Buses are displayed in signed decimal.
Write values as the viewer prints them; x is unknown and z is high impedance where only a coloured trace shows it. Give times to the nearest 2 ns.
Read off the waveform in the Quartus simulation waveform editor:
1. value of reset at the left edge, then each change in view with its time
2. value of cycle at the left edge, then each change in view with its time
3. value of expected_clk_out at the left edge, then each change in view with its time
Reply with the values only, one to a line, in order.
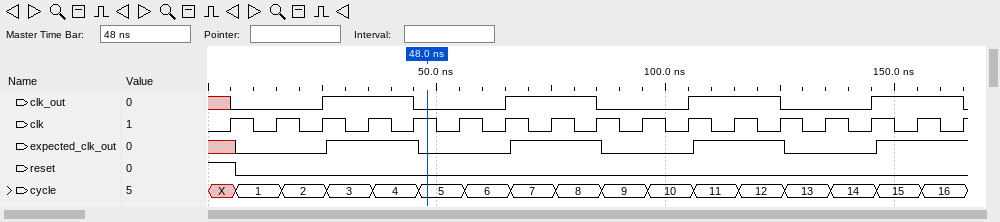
1, 0 at 6 ns
X, 1 at 6 ns, 2 at 16 ns, 3 at 26 ns, 4 at 36 ns, 5 at 46 ns, 6 at 56 ns, 7 at 66 ns, 8 at 76 ns, 9 at 86 ns, 10 at 96 ns, 11 at 106 ns, 12 at 116 ns, 13 at 126 ns, 14 at 136 ns, 15 at 146 ns, 16 at 156 ns
x, 0 at 6 ns, 1 at 26 ns, 0 at 46 ns, 1 at 66 ns, 0 at 86 ns, 1 at 106 ns, 0 at 126 ns, 1 at 146 ns
